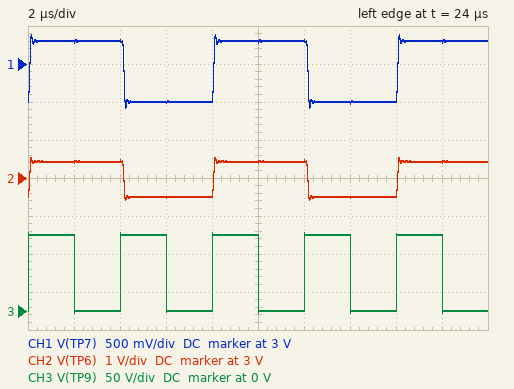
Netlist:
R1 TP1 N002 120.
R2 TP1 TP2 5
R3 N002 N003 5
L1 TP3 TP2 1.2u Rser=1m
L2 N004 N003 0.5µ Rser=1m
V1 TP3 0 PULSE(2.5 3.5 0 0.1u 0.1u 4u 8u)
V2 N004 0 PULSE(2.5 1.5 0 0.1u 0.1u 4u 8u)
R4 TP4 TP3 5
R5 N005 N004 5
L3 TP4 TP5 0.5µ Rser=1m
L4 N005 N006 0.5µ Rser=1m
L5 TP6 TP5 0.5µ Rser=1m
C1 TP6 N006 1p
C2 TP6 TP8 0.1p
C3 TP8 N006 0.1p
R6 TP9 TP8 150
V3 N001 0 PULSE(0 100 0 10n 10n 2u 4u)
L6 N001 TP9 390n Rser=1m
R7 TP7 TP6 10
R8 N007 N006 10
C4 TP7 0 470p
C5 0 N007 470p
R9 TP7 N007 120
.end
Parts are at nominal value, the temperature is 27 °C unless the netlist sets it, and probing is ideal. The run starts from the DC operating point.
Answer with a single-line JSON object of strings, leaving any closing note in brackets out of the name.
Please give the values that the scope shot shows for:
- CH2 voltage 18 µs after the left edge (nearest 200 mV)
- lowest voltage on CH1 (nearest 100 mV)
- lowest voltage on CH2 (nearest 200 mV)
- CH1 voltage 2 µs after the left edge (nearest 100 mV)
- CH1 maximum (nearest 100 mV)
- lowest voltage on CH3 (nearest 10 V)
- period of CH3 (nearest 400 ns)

{"CH2 voltage 18 µs after the left edge": "3.4 V", "lowest voltage on CH1": "2.4 V", "lowest voltage on CH2": "2.4 V", "CH1 voltage 2 µs after the left edge": "3.3 V", "CH1 maximum": "3.4 V", "lowest voltage on CH3": "0 V", "period of CH3": "4.0 µs"}
